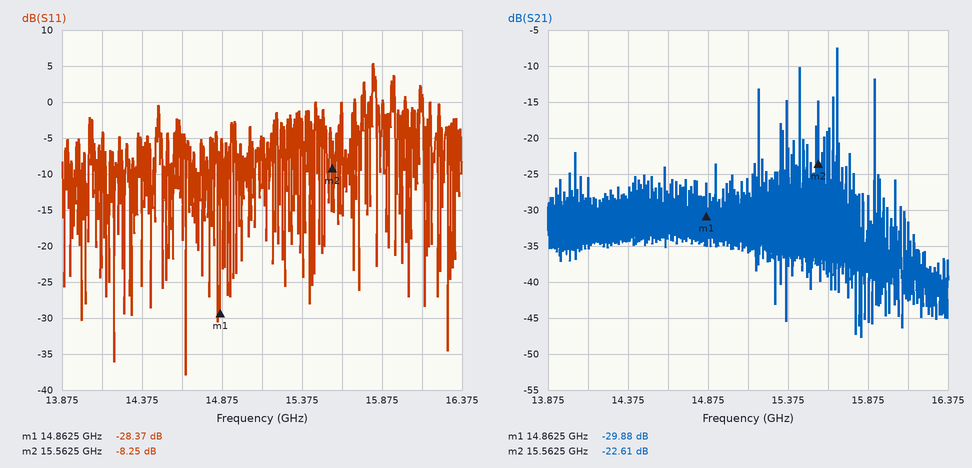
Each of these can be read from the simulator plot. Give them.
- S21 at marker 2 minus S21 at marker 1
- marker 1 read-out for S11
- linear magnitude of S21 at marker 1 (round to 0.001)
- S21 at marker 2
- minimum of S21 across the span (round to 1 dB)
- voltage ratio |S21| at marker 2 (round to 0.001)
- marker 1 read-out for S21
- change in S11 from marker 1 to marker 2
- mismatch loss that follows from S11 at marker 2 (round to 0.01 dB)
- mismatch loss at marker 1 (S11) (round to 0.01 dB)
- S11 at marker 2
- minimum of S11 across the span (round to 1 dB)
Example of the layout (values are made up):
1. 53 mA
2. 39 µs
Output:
1. 7.27 dB
2. -28.37 dB
3. 0.032
4. -22.61 dB
5. -48 dB
6. 0.074
7. -29.88 dB
8. 20.12 dB
9. 0.70 dB
10. 0.01 dB
11. -8.25 dB
12. -38 dB
